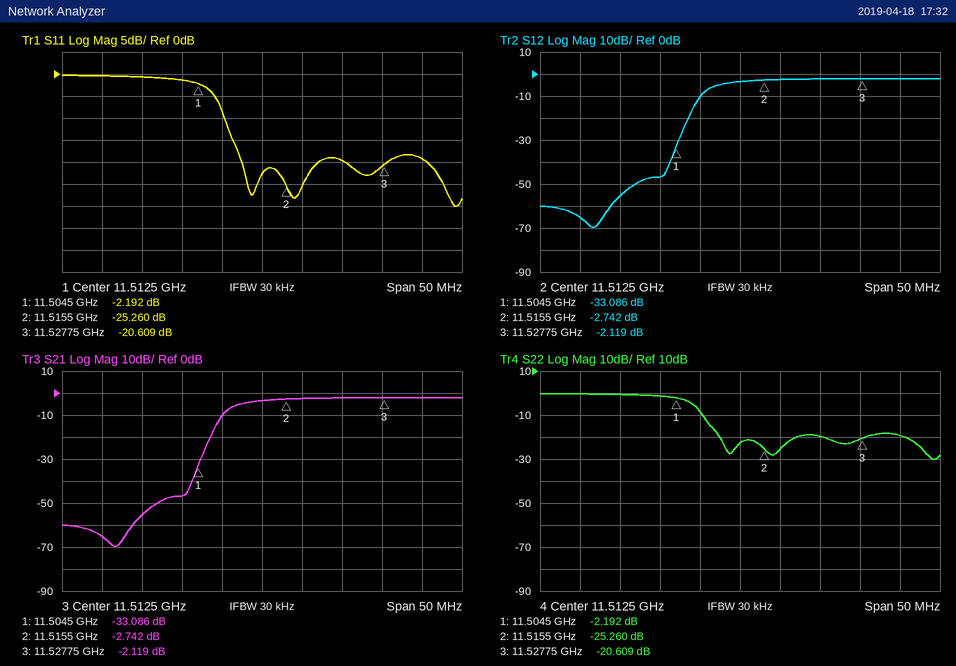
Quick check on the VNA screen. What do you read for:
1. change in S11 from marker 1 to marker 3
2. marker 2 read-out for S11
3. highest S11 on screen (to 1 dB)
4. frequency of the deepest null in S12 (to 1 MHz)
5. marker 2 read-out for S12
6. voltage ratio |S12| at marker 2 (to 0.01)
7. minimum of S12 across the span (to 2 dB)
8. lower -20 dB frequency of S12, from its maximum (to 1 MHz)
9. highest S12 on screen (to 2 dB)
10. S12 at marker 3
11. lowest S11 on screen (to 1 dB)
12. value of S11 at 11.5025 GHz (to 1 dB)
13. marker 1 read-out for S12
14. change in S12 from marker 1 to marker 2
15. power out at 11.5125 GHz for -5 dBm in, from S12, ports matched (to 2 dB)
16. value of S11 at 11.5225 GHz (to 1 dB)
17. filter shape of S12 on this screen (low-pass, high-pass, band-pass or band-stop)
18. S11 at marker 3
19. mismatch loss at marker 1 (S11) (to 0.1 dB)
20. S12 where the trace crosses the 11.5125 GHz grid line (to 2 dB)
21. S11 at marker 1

-18.417 dB
-25.260 dB
0 dB
11.494 GHz
-2.742 dB
0.73
-70 dB
11.506 GHz
-2 dB
-2.119 dB
-30 dB
-1 dB
-33.086 dB
30.344 dB
-8 dBm
-20 dB
high-pass
-20.609 dB
4.0 dB
-4 dB
-2.192 dB
